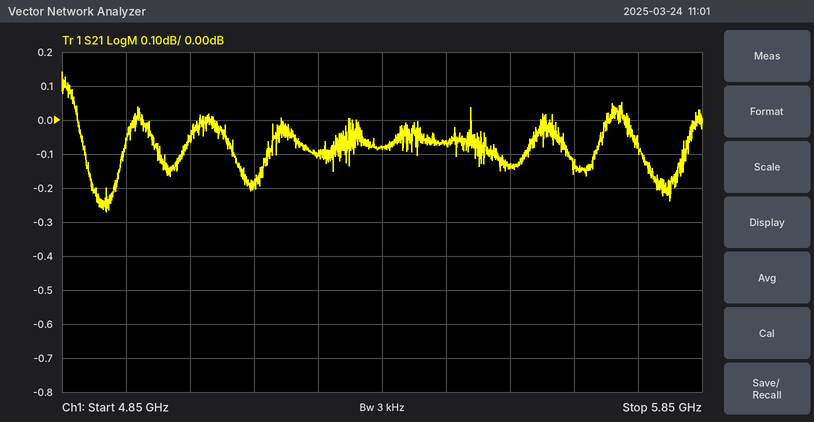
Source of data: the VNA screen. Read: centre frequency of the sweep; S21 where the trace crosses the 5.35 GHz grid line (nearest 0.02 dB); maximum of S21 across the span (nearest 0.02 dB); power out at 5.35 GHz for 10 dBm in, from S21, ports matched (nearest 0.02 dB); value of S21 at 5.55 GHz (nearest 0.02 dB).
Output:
5.35 GHz
-0.08 dB
0.14 dB
9.92 dBm
-0.14 dB
